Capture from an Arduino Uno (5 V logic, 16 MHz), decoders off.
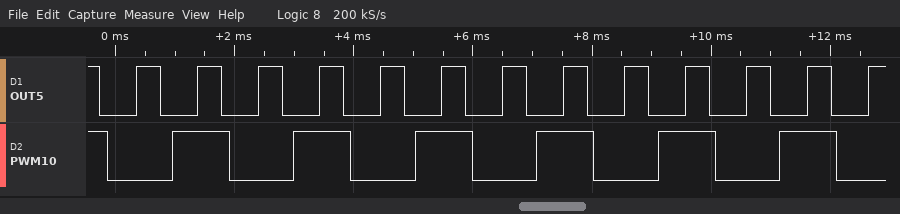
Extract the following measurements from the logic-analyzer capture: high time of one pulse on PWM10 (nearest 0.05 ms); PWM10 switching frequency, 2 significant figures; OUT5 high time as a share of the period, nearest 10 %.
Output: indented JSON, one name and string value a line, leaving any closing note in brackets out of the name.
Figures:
{
  "high time of one pulse on PWM10": "0.95 ms",
  "PWM10 switching frequency, 2 significant figures": "490 Hz",
  "OUT5 high time as a share of the period, nearest 10 %": "40 %"
}
